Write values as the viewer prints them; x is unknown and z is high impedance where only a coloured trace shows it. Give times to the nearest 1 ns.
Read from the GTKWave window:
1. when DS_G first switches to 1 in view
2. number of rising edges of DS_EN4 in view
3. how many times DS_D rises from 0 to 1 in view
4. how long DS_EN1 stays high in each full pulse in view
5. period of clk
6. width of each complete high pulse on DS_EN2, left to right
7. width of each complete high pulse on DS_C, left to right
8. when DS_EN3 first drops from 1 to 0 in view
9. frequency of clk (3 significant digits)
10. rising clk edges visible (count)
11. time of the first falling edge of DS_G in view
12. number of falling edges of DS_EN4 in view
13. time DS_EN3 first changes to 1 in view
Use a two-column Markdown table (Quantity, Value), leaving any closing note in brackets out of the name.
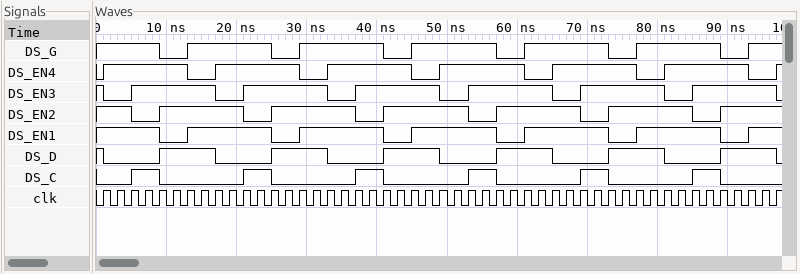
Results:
| Quantity | Value |
|---|---|
| when DS_G first switches to 1 in view | 13 ns |
| number of rising edges of DS_EN4 in view | 7 |
| how many times DS_D rises from 0 to 1 in view | 6 |
| how long DS_EN1 stays high in each full pulse in view | 12 ns, 12 ns, 12 ns, 12 ns, 12 ns |
| period of clk | 2 ns |
| width of each complete high pulse on DS_EN2, left to right | 12 ns, 12 ns, 12 ns, 12 ns, 12 ns |
| width of each complete high pulse on DS_C, left to right | 4 ns, 4 ns, 4 ns, 4 ns, 4 ns, 4 ns |
| when DS_EN3 first drops from 1 to 0 in view | 1 ns |
| frequency of clk | 500 MHz |
| rising clk edges visible | 49 |
| time of the first falling edge of DS_G in view | 9 ns |
| number of falling edges of DS_EN4 in view | 6 |
| time DS_EN3 first changes to 1 in view | 5 ns |
